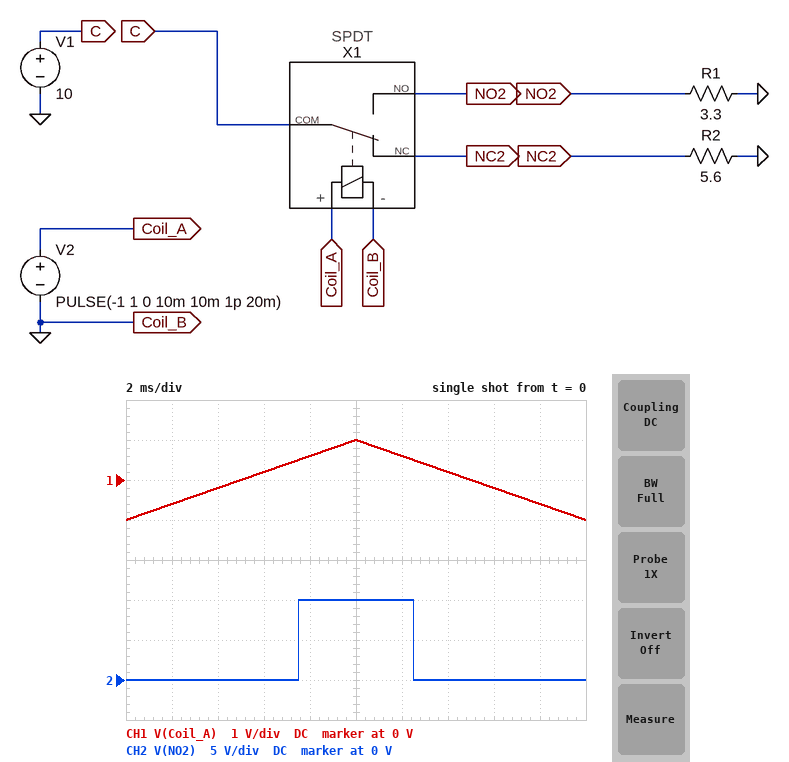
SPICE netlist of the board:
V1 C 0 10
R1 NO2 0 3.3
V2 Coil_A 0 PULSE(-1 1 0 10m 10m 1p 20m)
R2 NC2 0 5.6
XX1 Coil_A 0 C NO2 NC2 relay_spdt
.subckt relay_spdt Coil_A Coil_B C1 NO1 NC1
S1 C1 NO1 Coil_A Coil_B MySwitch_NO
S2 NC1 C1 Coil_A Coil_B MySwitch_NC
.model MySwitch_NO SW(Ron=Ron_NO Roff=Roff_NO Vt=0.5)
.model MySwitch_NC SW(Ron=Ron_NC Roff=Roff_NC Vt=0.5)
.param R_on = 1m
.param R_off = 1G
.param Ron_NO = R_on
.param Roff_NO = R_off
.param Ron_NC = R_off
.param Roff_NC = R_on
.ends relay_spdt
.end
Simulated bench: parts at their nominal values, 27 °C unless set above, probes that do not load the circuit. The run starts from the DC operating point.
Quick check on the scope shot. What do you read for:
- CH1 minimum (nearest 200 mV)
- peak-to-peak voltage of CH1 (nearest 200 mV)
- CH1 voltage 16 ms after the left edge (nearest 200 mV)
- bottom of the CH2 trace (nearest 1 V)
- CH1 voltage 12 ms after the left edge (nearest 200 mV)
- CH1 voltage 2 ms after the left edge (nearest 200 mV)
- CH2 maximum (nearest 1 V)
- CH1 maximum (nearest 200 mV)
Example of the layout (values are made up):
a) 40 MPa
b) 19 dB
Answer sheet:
a) -1.0 V
b) 2.0 V
c) -200 mV
d) 0 V
e) 600 mV
f) -600 mV
g) 10 V
h) 1.0 V
